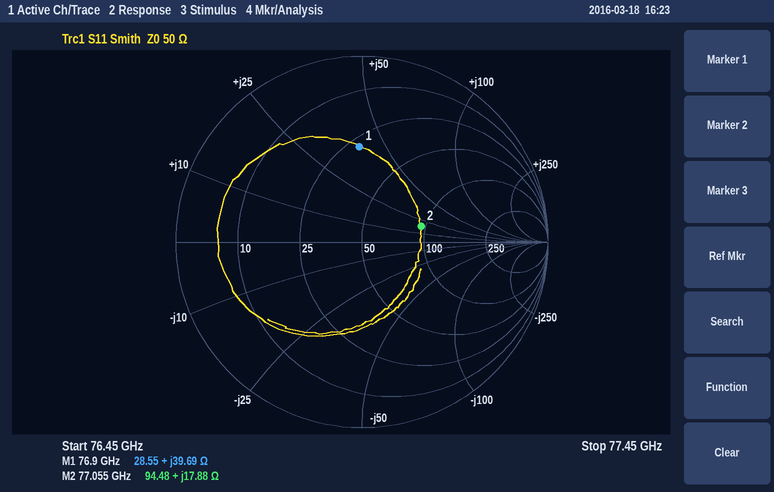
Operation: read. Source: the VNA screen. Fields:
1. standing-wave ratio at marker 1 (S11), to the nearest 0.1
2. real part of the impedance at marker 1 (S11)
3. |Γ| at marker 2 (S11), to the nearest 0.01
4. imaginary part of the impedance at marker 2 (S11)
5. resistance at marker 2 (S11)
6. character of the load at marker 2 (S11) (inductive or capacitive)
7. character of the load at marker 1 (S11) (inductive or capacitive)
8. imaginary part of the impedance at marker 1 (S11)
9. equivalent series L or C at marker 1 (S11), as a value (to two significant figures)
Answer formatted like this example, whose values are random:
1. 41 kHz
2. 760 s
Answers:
1. 3.1
2. 28.55 Ω
3. 0.33
4. +17.88 Ω
5. 94.48 Ω
6. inductive
7. inductive
8. +39.69 Ω
9. 82 pH
